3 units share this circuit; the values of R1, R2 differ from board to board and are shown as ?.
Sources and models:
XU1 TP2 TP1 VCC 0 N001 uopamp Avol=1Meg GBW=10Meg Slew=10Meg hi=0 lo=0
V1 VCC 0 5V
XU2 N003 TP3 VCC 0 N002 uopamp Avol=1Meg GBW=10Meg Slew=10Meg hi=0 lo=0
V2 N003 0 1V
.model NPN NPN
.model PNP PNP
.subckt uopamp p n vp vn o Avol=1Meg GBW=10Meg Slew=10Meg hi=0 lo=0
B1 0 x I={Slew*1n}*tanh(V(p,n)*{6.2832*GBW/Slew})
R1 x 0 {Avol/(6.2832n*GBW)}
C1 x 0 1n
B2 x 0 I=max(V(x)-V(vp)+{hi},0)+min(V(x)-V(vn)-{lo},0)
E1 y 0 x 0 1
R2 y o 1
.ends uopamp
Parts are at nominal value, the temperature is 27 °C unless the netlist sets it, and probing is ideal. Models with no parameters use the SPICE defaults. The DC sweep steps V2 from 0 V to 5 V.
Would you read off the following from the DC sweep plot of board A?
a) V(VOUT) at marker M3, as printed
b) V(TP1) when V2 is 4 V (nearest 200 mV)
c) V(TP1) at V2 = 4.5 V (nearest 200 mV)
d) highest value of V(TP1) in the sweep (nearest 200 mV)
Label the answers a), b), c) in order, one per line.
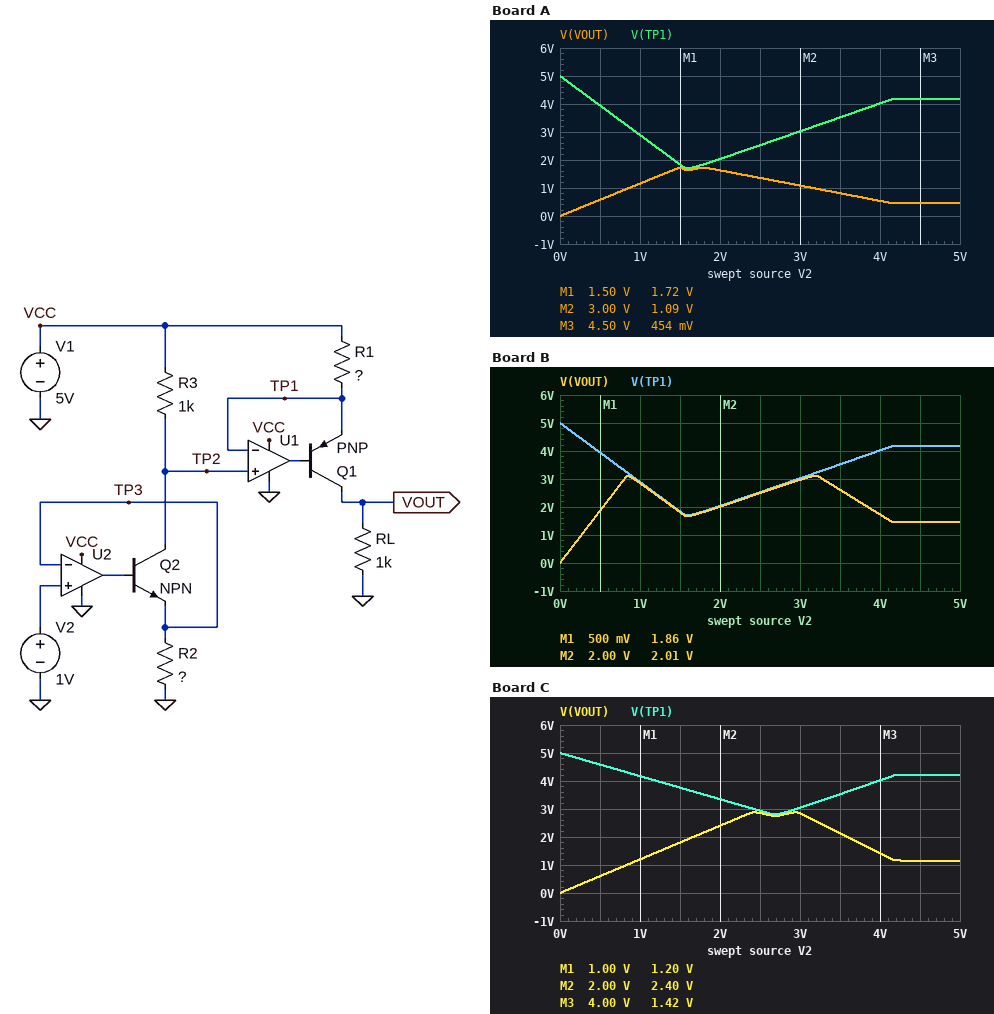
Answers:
a) 454 mV
b) 4.0 V
c) 4.2 V
d) 5.0 V
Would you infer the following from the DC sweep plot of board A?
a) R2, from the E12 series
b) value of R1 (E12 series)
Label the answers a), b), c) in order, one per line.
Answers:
a) 470 Ω
b) 1.8 kΩ
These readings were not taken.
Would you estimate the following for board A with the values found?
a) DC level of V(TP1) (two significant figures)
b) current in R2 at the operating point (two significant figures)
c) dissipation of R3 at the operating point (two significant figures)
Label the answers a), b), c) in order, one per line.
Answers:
a) 2.9 V
b) 2.1 mA
c) 4.4 mW
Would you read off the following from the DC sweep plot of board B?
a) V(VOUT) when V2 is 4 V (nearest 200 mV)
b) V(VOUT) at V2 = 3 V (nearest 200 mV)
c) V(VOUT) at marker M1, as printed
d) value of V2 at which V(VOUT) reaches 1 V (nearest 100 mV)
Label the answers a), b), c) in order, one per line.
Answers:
a) 1.8 V
b) 3.0 V
c) 1.86 V
d) 300 mV
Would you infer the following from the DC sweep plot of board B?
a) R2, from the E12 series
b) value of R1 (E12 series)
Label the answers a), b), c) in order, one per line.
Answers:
a) 470 Ω
b) 560 Ω
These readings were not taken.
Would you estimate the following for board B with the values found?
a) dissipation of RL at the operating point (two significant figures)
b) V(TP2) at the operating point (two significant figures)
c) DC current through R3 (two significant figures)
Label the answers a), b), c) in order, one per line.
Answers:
a) 8.1 mW
b) 2.9 V
c) 2.1 mA
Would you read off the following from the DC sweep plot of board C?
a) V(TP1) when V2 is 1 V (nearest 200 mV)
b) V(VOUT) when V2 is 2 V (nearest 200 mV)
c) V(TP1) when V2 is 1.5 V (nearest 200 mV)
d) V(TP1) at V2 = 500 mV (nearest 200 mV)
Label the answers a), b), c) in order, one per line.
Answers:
a) 4.2 V
b) 2.4 V
c) 3.8 V
d) 4.6 V
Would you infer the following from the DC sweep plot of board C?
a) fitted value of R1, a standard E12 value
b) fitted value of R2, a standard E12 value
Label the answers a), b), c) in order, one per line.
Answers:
a) 680 Ω
b) 1.2 kΩ
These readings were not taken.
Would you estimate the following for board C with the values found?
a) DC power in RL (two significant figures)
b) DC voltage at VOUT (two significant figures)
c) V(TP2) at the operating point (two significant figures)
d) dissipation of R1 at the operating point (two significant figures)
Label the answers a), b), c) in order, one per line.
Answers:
a) 1.4 mW
b) 1.2 V
c) 4.2 V
d) 1.0 mW
